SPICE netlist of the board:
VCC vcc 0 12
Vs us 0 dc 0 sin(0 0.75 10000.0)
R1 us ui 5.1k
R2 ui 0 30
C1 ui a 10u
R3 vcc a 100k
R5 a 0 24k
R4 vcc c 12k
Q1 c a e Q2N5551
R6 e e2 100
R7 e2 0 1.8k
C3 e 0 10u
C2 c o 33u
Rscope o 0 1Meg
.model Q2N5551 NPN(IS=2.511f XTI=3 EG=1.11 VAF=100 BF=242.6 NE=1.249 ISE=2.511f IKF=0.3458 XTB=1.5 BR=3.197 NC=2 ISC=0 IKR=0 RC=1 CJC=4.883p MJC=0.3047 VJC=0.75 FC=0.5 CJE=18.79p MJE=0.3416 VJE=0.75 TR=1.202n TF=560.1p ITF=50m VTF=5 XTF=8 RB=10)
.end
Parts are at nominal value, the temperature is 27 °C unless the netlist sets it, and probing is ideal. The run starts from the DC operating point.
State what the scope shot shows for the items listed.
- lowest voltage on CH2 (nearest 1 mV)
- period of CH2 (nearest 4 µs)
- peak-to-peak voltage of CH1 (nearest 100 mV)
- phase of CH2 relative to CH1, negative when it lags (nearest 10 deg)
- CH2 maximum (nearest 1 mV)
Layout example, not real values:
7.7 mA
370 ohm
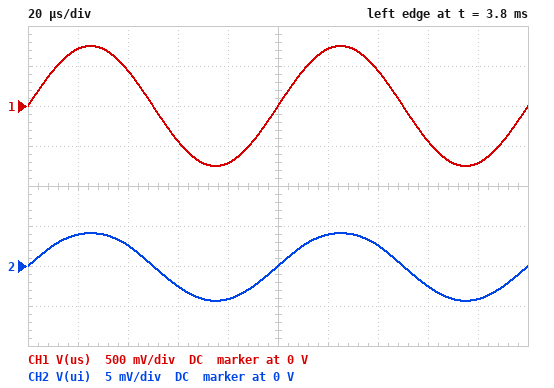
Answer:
-4 mV
100 µs
1.5 V
0 deg
4 mV
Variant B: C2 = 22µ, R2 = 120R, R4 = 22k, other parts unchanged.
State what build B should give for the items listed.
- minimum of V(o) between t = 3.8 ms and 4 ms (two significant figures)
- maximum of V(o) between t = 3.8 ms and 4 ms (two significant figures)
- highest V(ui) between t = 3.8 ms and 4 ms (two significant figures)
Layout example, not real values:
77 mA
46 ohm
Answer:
-27 mV
2.4 V
9.3 mV
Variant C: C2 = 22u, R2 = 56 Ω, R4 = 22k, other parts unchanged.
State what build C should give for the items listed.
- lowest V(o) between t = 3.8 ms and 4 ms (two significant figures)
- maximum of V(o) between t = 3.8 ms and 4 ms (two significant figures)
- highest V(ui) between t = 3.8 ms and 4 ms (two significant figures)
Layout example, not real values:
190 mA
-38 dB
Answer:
-16 mV
420 mV
6.1 mV
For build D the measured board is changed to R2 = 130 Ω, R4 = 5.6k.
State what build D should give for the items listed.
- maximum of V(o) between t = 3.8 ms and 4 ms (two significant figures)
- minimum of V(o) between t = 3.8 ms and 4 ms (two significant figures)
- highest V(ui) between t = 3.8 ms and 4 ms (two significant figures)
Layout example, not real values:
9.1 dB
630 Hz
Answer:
2.4 V
-3.2 V
18 mV
